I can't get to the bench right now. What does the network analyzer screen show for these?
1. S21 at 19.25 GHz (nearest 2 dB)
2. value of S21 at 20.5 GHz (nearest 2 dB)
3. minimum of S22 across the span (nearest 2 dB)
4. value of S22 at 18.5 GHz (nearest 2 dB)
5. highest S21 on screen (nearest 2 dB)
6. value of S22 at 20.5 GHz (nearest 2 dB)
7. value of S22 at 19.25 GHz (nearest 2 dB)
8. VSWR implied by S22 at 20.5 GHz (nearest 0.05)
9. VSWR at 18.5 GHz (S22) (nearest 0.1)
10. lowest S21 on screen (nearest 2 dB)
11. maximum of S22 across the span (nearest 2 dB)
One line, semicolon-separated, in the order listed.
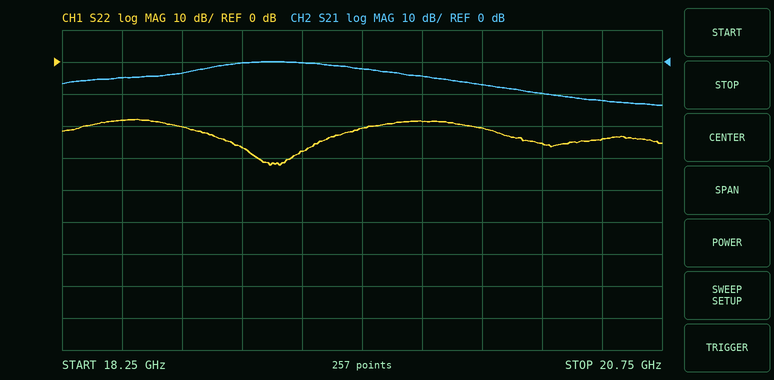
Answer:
0 dB; -12 dB; -32 dB; -18 dB; 0 dB; -24 dB; -28 dB; 1.15; 1.3; -14 dB; -18 dB
